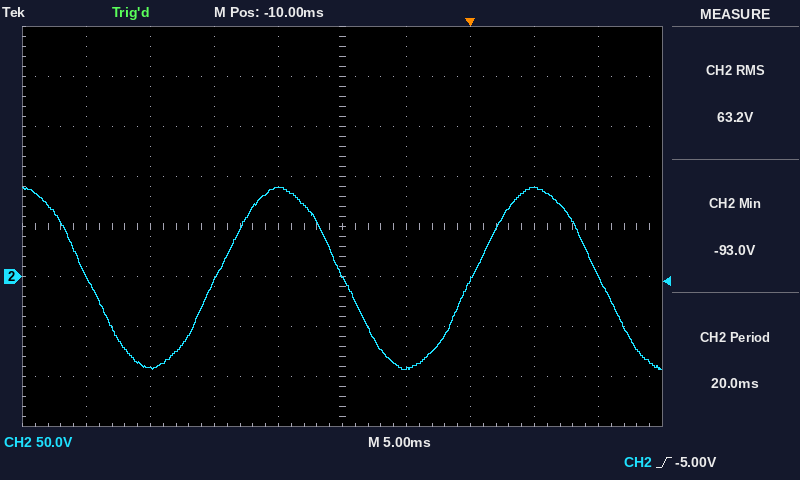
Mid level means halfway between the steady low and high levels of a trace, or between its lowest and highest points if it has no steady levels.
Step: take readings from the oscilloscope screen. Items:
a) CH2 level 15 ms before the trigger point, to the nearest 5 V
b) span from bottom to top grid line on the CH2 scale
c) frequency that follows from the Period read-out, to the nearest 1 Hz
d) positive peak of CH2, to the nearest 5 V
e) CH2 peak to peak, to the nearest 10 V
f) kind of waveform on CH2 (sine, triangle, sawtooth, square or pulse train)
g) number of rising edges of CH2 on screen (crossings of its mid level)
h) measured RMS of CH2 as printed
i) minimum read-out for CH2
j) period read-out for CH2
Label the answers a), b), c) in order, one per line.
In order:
a) 90 V
b) 400 V
c) 50 Hz
d) 90 V
e) 180 V
f) sine
g) 2
h) 63.2 V
i) -93.0 V
j) 20.0 ms
